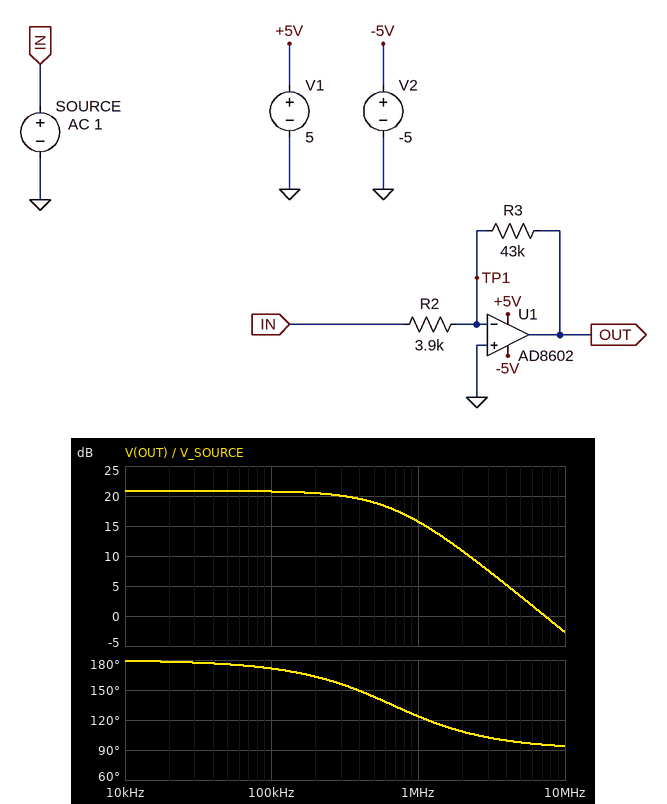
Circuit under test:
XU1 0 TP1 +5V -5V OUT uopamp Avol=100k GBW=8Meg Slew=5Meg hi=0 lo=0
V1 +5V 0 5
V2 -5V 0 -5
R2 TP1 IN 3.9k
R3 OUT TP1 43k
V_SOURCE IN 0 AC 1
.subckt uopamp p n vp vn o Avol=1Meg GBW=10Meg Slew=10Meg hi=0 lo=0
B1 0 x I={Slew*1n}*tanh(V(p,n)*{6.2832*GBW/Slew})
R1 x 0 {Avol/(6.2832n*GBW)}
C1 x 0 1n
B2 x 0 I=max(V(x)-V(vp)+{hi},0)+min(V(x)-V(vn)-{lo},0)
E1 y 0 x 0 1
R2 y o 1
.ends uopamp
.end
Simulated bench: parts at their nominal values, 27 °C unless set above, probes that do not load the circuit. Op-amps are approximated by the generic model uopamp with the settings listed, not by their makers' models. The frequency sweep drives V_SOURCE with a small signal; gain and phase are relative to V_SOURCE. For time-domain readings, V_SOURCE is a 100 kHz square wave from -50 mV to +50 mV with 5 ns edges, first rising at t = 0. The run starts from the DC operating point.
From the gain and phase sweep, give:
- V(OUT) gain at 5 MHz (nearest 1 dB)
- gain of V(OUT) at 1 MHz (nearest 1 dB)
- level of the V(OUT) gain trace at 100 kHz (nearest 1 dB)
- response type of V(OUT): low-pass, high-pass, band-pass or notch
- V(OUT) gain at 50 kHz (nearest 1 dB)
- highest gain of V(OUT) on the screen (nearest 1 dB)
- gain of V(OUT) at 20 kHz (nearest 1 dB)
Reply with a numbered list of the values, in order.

1. 3 dB
2. 16 dB
3. 21 dB
4. low-pass
5. 21 dB
6. 21 dB
7. 21 dB
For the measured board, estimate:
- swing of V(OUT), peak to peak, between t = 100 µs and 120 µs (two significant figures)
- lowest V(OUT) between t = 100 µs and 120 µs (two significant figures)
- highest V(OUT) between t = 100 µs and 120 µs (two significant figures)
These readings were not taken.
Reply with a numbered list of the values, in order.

1. 1.1 V
2. -550 mV
3. 550 mV
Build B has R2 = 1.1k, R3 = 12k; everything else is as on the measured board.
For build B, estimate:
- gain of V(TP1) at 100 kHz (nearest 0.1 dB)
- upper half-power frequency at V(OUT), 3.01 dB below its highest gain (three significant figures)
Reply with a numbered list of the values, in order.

1. -17.4 dB
2. 672 kHz
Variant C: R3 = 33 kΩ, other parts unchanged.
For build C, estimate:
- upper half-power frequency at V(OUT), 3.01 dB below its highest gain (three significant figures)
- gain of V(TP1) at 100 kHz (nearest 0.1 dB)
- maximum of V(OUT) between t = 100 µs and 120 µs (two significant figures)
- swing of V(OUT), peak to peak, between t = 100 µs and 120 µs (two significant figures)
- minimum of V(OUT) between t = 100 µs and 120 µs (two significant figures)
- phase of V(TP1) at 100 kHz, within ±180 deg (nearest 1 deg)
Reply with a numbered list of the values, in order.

1. 846 kHz
2. -19.6 dB
3. 420 mV
4. 850 mV
5. -420 mV
6. 83 deg
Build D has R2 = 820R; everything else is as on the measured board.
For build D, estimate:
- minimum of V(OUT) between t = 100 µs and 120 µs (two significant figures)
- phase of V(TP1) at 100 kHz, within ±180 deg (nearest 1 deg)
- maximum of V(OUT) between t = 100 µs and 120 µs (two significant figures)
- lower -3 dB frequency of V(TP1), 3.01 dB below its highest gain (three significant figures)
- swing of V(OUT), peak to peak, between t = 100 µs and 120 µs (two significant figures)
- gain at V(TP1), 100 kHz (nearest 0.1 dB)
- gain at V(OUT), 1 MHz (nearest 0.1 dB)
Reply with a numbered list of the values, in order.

1. -2.6 V
2. 56 deg
3. 2.6 V
4. 150 kHz
5. 5.1 V
6. -5.3 dB
7. 17.8 dB
